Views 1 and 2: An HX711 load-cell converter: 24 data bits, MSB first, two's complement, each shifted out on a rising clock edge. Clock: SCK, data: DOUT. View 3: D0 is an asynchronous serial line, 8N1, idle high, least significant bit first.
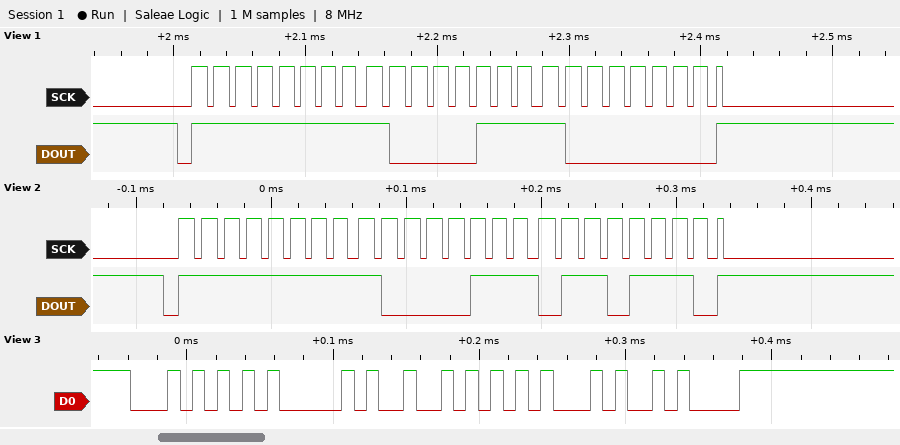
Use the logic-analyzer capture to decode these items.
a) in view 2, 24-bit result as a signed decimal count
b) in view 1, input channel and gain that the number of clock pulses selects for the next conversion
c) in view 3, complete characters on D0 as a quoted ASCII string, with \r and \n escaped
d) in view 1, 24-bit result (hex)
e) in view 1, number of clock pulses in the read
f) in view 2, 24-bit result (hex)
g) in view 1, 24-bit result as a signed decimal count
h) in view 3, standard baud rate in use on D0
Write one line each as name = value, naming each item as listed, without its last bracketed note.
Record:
in view 2, 24-bit result as a signed decimal count = -30866
in view 1, input channel and gain that the number of clock pulses selects for the next conversion = channel A, gain 128
in view 3, complete characters on D0 as a quoted ASCII string, with \r and \n escaped = "TARE\n"
in view 1, 24-bit result = 0xFF8780
in view 1, number of clock pulses in the read = 25
in view 2, 24-bit result = 0xFF876E
in view 1, 24-bit result as a signed decimal count = -30848
in view 3, standard baud rate in use on D0 = 115200 baud
